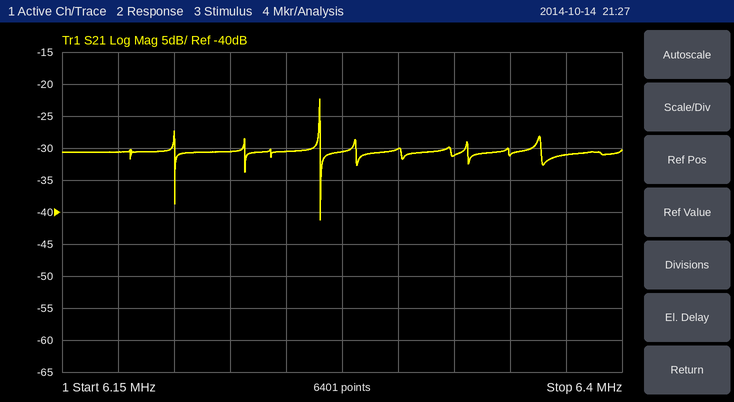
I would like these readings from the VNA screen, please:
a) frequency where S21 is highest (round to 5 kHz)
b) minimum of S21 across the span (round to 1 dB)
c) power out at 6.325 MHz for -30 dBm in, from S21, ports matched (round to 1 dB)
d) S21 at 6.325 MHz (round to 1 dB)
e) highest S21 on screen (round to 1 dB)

6.265 MHz
-41 dB
-61 dBm
-31 dB
-22 dB
